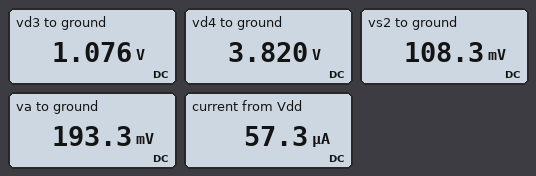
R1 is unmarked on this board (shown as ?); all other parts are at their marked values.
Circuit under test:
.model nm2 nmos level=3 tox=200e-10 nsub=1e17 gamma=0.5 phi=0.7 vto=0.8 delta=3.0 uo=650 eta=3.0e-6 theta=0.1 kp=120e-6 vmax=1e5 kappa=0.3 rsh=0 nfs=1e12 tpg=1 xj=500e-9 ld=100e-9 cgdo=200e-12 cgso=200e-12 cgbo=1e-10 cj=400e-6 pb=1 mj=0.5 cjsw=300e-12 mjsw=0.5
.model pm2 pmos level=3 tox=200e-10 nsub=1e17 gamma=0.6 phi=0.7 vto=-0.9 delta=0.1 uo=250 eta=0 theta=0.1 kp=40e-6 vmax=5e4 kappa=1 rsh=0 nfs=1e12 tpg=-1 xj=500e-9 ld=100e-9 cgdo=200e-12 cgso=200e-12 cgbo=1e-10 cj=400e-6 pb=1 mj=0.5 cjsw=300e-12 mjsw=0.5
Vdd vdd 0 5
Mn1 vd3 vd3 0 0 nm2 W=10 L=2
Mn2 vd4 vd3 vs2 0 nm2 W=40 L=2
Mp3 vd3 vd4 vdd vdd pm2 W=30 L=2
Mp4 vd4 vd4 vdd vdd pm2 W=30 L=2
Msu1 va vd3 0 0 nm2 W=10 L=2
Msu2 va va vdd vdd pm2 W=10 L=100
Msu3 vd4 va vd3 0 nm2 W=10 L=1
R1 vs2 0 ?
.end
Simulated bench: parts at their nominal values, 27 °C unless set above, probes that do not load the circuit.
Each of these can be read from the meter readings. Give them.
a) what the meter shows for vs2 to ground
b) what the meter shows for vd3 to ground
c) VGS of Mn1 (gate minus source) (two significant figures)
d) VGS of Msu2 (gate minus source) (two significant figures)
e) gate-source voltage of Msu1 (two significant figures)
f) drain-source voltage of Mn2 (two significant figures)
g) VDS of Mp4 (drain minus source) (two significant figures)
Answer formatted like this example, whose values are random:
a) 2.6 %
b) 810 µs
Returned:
a) 108.3 mV
b) 1.076 V
c) 1.1 V
d) -4.8 V
e) 1.1 V
f) 3.7 V
g) -1.2 V
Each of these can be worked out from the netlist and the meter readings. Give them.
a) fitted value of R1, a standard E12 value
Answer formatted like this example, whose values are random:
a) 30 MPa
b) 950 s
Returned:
a) 5.6 kΩ
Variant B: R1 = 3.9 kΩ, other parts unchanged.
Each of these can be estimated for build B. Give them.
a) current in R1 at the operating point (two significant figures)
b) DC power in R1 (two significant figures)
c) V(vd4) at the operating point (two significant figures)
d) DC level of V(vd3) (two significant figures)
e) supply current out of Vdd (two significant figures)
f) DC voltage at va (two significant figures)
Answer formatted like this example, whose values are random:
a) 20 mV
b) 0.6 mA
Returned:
a) 41 µA
b) 6.6 µW
c) 3.7 V
d) 1.2 V
e) 100 µA
f) 96 mV
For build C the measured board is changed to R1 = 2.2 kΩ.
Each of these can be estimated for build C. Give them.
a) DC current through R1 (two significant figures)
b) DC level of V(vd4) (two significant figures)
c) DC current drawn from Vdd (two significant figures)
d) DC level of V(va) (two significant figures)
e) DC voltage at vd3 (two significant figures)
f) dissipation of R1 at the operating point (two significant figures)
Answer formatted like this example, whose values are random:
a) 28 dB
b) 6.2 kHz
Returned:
a) 140 µA
b) 3.3 V
c) 300 µA
d) 49 mV
e) 1.6 V
f) 43 µW
